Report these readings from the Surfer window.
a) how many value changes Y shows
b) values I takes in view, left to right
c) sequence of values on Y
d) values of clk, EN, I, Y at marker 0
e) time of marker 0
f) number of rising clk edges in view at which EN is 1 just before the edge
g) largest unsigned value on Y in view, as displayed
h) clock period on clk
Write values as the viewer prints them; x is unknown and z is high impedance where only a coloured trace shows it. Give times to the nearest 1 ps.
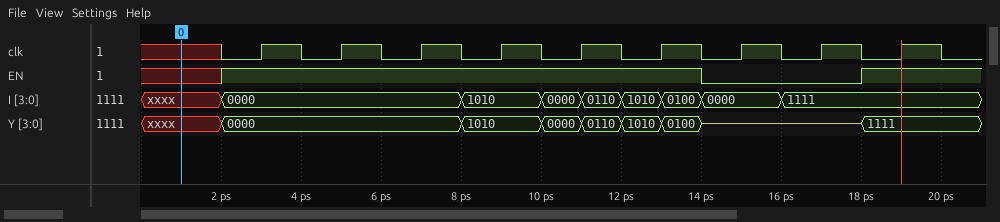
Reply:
8
xxxx, 0000, 1010, 0000, 0110, 1010, 0100, 0000, 1111
xxxx, 0000, 1010, 0000, 0110, 1010, 0100, z, 1111
clk=x, EN=x, I=xxxx, Y=xxxx
1 ps
7
1111
2 ps
